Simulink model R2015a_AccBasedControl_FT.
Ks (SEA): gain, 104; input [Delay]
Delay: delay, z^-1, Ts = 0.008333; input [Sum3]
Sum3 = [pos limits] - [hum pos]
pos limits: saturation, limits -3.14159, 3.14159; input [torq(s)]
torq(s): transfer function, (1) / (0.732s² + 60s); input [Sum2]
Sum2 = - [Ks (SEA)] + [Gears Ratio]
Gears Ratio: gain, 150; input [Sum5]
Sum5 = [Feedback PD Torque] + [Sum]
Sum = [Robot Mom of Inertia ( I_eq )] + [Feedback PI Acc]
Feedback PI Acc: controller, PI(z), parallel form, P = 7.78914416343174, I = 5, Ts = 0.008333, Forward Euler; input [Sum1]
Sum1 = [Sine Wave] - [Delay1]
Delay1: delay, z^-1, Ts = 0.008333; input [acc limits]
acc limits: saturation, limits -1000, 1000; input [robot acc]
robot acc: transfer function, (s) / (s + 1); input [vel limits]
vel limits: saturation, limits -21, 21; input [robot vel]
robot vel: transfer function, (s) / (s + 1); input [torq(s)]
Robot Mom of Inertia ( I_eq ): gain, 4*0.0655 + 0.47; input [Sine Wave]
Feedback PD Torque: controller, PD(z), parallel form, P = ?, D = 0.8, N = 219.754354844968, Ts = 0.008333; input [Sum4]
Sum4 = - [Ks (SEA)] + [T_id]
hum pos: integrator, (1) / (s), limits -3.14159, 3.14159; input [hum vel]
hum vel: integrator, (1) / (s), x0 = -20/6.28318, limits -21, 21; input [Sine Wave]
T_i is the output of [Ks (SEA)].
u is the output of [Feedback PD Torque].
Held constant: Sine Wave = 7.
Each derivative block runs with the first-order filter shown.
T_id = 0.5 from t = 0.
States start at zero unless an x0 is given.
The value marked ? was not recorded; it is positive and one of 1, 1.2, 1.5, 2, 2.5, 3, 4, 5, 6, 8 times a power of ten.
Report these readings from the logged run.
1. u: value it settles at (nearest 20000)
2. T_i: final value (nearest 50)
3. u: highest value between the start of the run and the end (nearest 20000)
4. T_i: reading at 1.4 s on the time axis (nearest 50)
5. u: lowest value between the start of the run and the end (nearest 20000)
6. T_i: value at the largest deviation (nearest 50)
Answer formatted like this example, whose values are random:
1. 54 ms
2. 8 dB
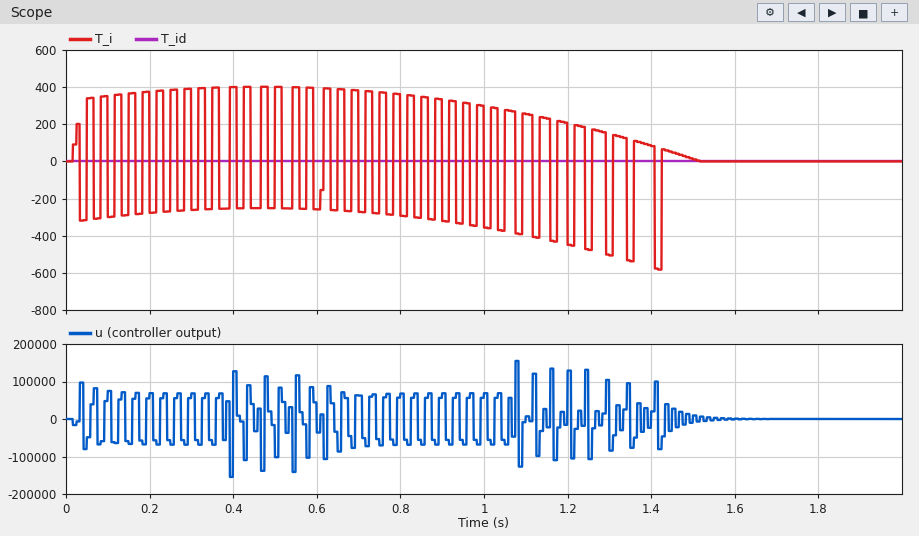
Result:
1. 0
2. 0
3. 160000
4. 100
5. -160000
6. -600
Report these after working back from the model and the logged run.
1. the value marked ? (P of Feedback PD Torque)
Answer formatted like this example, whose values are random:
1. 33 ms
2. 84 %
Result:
1. 1.5
